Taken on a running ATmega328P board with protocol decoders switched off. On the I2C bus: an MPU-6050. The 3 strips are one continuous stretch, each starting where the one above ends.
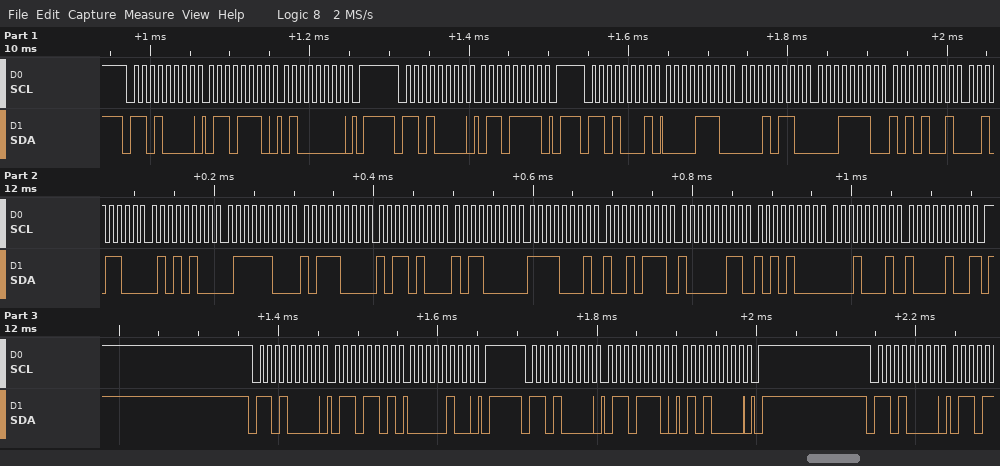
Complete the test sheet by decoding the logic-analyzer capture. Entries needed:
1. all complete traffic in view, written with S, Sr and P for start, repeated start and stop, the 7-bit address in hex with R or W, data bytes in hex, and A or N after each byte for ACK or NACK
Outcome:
S 68W A 6E A 40 A P S 68W A 6F A P S 68R A 0E A 16 A 1E A A9 A 2C A 54 A 7C A B8 A B4 A B0 A F1 A 97 A 83 A A8 A 11 A 84 N P S 68W A 6D A 04 A P S 68W A 6E A 50 A P S 68W A
